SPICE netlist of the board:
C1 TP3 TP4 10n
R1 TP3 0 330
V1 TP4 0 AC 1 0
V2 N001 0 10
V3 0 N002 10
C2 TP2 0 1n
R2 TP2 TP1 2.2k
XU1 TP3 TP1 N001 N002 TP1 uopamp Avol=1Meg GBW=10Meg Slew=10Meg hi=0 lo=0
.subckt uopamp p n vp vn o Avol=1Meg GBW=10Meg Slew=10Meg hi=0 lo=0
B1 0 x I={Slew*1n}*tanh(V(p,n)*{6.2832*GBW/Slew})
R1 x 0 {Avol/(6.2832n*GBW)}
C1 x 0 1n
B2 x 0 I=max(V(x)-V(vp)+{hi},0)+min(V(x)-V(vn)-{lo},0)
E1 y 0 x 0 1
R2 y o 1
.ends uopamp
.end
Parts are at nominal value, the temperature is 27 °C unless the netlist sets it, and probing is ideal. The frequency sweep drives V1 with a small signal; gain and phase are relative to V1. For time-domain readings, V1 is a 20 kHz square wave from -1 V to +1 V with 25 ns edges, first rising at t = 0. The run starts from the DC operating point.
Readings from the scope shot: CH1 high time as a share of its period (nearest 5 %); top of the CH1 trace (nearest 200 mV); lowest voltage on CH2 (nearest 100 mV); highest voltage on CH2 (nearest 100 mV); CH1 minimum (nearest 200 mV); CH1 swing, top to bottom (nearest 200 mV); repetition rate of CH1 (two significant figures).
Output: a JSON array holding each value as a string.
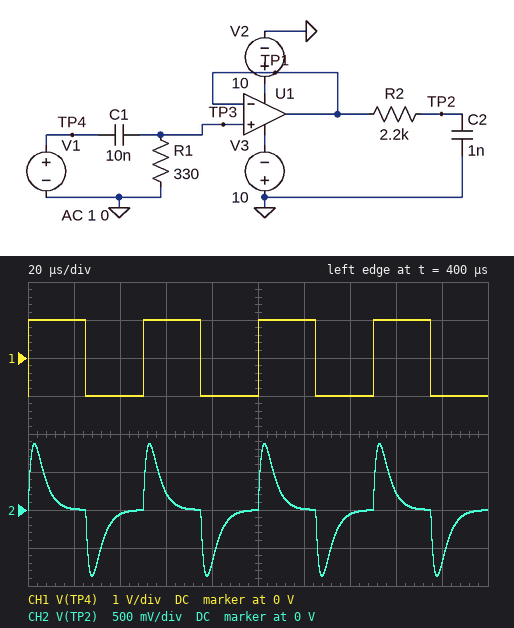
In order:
["50 %", "1.0 V", "-900 mV", "900 mV", "-1.0 V", "2.0 V", "20 kHz"]
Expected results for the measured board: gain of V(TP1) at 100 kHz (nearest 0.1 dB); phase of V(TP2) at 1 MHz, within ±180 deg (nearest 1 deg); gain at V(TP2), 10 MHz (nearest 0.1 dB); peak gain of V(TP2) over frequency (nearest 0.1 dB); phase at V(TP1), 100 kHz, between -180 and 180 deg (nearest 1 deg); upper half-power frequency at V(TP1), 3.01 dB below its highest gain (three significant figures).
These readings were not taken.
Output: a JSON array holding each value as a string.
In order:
["-0.9 dB", "-89 deg", "-45.8 dB", "-4.4 dB", "25 deg", "10.1 MHz"]
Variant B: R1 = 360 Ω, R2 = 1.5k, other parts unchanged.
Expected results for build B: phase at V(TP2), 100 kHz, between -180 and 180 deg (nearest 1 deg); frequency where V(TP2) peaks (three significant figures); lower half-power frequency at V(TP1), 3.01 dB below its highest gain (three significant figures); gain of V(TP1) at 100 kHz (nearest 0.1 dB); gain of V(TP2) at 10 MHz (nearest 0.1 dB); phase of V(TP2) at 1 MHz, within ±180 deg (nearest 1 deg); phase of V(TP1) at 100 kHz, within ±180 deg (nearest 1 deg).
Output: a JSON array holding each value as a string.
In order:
["-20 deg", "68.5 kHz", "43.8 kHz", "-0.8 dB", "-42.5 dB", "-87 deg", "23 deg"]
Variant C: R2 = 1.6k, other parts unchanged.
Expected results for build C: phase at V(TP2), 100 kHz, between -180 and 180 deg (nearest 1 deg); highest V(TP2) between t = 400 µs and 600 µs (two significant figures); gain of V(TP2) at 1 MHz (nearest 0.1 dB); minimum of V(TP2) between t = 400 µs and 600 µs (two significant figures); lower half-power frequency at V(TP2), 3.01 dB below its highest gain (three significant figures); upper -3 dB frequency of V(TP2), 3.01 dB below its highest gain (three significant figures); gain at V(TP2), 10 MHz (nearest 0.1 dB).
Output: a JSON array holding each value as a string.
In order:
["-20 deg", "990 mV", "-20.1 dB", "-990 mV", "27.4 kHz", "175 kHz", "-43.1 dB"]
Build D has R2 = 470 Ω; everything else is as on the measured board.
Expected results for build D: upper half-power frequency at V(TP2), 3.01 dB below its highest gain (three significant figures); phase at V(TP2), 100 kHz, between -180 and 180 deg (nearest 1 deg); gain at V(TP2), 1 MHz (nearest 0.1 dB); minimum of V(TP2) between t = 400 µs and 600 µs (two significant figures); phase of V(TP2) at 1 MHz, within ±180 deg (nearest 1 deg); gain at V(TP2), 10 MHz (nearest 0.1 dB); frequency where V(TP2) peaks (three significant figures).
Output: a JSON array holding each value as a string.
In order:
["425 kHz", "9 deg", "-9.9 dB", "-1.4 V", "-74 deg", "-32.4 dB", "128 kHz"]
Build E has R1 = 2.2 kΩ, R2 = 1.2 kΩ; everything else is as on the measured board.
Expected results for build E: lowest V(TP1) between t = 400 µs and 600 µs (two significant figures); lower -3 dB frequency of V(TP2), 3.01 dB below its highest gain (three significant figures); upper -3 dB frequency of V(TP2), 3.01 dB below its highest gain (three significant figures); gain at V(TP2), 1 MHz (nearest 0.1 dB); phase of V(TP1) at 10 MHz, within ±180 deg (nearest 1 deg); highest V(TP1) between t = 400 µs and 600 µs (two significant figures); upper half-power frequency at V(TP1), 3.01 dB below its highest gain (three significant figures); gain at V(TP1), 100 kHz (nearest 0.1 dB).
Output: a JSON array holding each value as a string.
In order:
["-1.5 V", "6.55 kHz", "146 kHz", "-17.7 dB", "-45 deg", "1.5 V", "10.0 MHz", "0 dB"]
